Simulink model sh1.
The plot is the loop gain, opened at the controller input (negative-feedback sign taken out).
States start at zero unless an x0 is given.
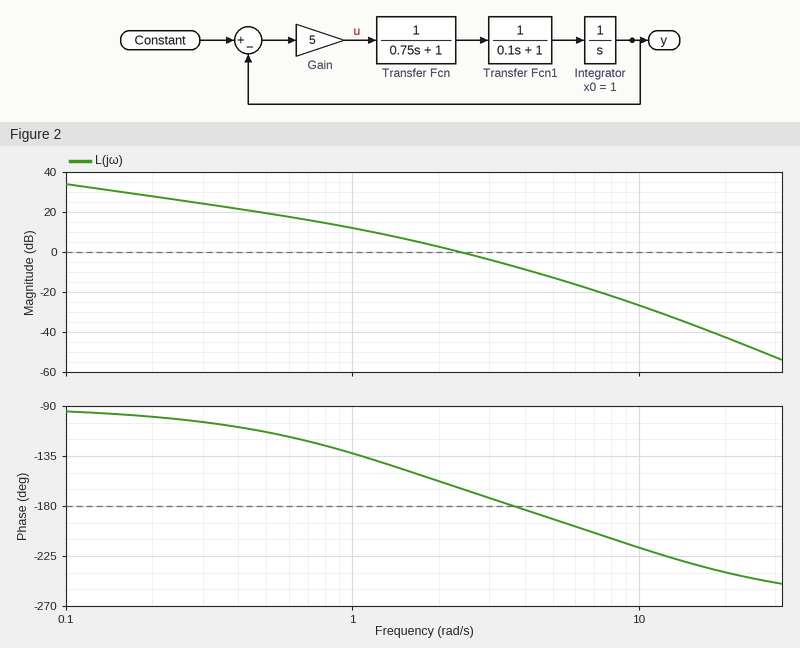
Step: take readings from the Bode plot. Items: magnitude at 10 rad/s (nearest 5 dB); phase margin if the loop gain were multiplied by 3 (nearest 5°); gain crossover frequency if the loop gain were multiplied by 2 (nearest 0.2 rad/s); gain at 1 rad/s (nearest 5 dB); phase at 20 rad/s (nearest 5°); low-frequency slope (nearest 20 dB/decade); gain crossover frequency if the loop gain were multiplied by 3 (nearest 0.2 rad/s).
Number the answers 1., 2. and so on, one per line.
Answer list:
1. -25 dB
2. -5°
3. 3.4 rad/s
4. 10 dB
5. -240°
6. -20 dB/decade
7. 4.2 rad/s
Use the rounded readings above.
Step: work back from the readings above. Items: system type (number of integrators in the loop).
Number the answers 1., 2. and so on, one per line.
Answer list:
1. 1
